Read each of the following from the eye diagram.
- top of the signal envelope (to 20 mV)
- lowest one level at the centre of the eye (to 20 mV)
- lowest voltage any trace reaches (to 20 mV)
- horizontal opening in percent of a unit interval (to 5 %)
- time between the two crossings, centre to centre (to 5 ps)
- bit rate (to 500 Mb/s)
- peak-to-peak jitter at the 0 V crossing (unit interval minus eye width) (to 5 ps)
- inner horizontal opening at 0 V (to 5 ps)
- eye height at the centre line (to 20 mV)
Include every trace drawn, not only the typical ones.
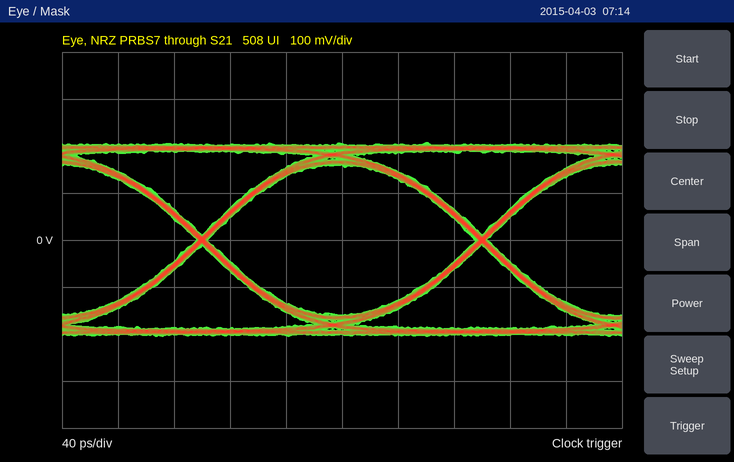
200 mV
160 mV
-200 mV
95 %
200 ps
5.0 Gb/s
10 ps
190 ps
320 mV
